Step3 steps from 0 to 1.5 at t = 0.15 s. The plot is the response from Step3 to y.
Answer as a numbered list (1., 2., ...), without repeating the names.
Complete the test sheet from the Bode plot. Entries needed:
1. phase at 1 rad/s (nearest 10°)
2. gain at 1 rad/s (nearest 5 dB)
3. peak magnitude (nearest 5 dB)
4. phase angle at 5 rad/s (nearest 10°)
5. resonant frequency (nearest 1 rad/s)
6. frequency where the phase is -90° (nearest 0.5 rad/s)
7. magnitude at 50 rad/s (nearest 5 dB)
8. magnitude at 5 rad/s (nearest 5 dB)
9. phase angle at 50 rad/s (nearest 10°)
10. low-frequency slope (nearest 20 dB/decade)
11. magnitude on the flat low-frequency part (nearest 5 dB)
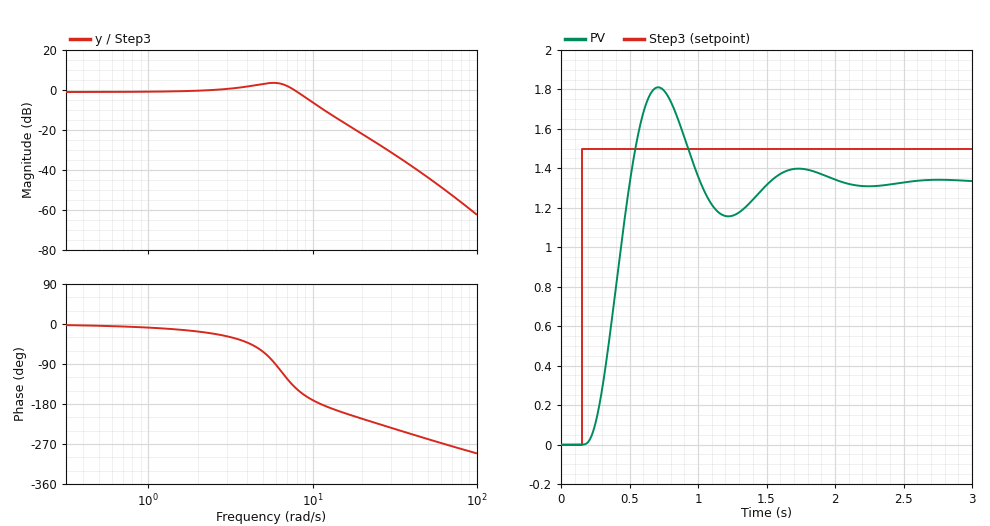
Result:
1. -10°
2. 0 dB
3. 5 dB
4. -60°
5. 6 rad/s
6. 6.0 rad/s
7. -45 dB
8. 5 dB
9. -260°
10. 0 dB/decade
11. 0 dB
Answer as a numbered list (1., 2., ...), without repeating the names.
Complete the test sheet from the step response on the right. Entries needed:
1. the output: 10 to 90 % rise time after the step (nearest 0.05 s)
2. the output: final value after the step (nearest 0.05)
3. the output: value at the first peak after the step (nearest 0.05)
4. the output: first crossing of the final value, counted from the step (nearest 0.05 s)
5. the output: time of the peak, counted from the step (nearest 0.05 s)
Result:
1. 0.20 s
2. 1.35
3. 1.80
4. 0.35 s
5. 0.55 s
